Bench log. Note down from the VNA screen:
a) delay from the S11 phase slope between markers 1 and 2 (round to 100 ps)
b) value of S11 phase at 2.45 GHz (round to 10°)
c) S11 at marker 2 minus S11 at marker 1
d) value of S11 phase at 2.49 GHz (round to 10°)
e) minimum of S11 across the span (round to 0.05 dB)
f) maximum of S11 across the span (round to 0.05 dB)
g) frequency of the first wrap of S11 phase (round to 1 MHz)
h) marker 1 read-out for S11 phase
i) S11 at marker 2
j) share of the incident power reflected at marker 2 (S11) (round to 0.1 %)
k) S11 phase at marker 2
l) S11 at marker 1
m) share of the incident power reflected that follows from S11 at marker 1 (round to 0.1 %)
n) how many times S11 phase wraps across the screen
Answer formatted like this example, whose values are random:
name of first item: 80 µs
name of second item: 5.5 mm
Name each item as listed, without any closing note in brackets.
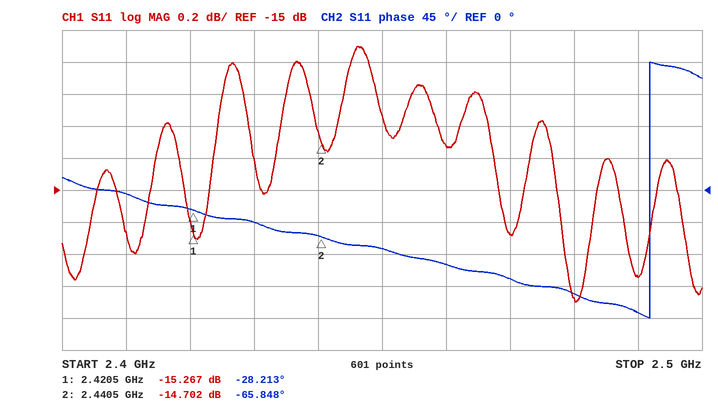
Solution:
delay from the S11 phase slope between markers 1 and 2: 5.2 ns
value of S11 phase at 2.45 GHz: -80°
S11 at marker 2 minus S11 at marker 1: 0.565 dB
value of S11 phase at 2.49 GHz: -170°
minimum of S11 across the span: -15.70 dB
maximum of S11 across the span: -14.10 dB
frequency of the first wrap of S11 phase: 2.492 GHz
marker 1 read-out for S11 phase: -28.213°
S11 at marker 2: -14.702 dB
share of the incident power reflected at marker 2 (S11): 3.4 %
S11 phase at marker 2: -65.848°
S11 at marker 1: -15.267 dB
share of the incident power reflected that follows from S11 at marker 1: 3.0 %
how many times S11 phase wraps across the screen: 1
